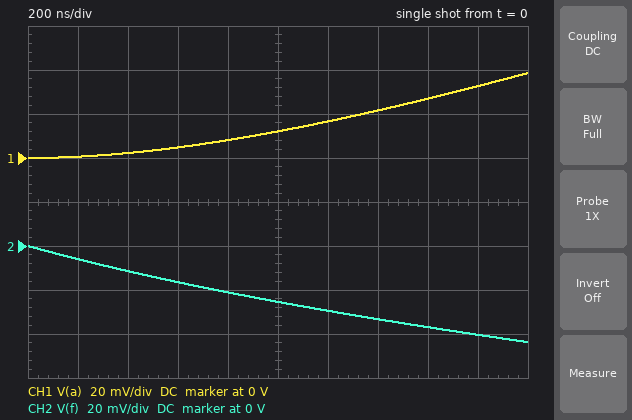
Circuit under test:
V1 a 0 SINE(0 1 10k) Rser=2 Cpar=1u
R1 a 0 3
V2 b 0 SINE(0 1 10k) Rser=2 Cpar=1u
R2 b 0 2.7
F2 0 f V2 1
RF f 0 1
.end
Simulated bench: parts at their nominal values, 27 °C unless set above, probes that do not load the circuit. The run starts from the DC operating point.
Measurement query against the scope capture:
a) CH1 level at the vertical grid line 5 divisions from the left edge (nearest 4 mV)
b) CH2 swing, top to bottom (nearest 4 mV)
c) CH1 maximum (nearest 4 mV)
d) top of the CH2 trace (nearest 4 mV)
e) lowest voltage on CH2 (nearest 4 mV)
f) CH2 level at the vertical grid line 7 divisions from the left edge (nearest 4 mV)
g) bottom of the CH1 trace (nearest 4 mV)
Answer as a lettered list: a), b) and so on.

a) 12 mV
b) 44 mV
c) 40 mV
d) 0 V
e) -44 mV
f) -32 mV
g) 0 V
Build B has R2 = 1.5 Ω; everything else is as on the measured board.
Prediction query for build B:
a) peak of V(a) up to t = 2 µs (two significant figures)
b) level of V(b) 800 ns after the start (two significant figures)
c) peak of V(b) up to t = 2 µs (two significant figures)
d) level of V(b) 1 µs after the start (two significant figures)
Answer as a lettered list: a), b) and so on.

a) 39 mV
b) 7.5 mV
c) 33 mV
d) 11 mV
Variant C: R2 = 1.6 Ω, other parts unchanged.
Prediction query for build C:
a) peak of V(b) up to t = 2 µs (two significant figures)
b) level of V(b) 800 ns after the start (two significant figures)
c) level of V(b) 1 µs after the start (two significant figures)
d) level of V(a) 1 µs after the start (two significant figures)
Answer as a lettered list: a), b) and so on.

a) 34 mV
b) 7.6 mV
c) 11 mV
d) 12 mV
